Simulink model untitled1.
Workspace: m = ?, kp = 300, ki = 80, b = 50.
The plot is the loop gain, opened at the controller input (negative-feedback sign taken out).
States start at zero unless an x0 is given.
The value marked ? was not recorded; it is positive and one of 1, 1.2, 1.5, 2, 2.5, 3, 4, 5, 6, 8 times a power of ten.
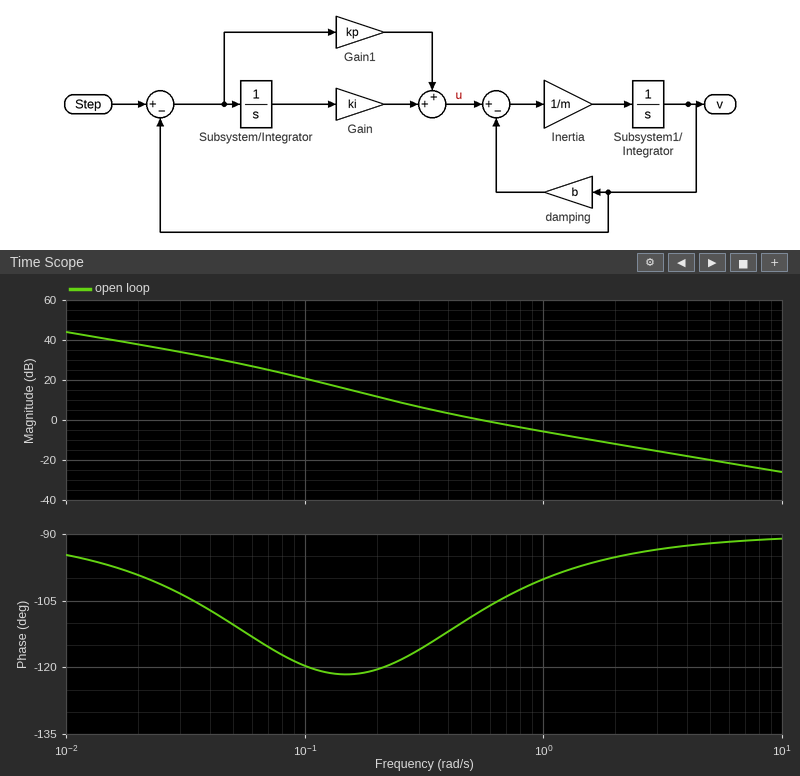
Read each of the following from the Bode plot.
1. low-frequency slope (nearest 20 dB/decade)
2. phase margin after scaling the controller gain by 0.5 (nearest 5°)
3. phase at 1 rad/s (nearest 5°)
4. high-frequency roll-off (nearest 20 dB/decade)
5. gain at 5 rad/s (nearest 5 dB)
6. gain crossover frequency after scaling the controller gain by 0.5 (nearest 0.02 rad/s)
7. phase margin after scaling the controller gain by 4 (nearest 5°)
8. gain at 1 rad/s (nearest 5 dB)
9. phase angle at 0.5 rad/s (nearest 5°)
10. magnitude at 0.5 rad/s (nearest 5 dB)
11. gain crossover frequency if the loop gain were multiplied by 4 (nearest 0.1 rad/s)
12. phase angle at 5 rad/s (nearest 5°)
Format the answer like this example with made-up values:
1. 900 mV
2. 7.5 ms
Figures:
1. -20 dB/decade
2. 65°
3. -100°
4. -20 dB/decade
5. -20 dB
6. 0.32 rad/s
7. 85°
8. -5 dB
9. -110°
10. 0 dB
11. 2.0 rad/s
12. -90°
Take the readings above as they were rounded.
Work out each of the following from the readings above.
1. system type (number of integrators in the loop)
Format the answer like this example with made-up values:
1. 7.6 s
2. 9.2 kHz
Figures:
1. 1
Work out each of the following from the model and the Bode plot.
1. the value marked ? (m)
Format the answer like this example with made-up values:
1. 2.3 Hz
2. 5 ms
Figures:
1. 600
